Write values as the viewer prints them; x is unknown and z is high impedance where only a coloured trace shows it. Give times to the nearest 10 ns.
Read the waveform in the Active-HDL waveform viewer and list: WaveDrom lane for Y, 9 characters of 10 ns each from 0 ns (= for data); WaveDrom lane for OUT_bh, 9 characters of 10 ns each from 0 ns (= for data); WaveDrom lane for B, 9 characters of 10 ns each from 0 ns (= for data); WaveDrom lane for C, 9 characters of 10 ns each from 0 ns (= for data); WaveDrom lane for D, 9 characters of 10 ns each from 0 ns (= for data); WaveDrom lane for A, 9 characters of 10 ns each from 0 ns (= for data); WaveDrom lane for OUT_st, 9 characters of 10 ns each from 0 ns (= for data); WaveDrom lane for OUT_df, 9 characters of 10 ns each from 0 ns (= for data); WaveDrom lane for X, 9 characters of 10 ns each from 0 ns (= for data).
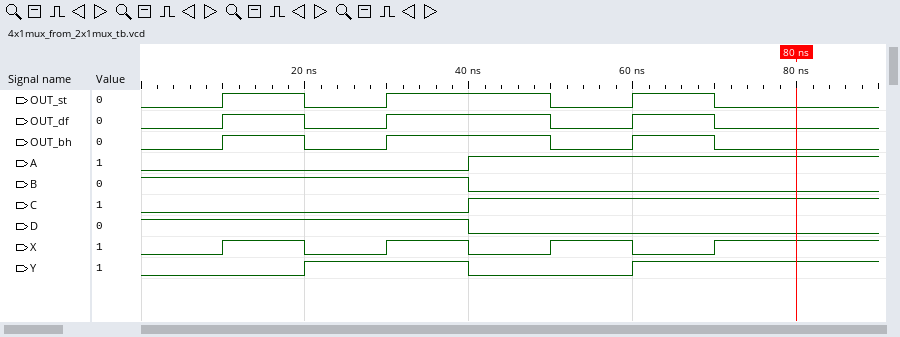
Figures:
{name: 'Y', wave: '0.1.0.1..'}
{name: 'OUT_bh', wave: '0101.010.'}
{name: 'B', wave: '1...0....'}
{name: 'C', wave: '0...1....'}
{name: 'D', wave: '1...0....'}
{name: 'A', wave: '0...1....'}
{name: 'OUT_st', wave: '0101.010.'}
{name: 'OUT_df', wave: '0101.010.'}
{name: 'X', wave: '01010101.'}
